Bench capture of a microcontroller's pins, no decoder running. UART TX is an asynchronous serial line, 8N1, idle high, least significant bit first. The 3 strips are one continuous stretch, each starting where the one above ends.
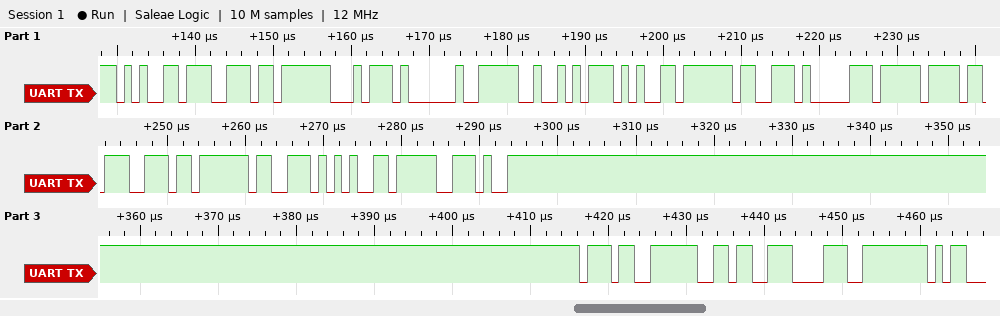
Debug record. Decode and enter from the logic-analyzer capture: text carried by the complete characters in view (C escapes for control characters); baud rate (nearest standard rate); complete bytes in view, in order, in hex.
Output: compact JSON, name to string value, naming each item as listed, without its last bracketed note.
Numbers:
{"text carried by the complete characters in view": "\"ent Response.768\"", "baud rate": "1000000 baud", "complete bytes in view, in order, in hex": "0x65 0x6E 0x74 0x20 0x52 0x65 0x73 0x70 0x6F 0x6E 0x73 0x65 0x2E 0x37 0x36 0x38"}
